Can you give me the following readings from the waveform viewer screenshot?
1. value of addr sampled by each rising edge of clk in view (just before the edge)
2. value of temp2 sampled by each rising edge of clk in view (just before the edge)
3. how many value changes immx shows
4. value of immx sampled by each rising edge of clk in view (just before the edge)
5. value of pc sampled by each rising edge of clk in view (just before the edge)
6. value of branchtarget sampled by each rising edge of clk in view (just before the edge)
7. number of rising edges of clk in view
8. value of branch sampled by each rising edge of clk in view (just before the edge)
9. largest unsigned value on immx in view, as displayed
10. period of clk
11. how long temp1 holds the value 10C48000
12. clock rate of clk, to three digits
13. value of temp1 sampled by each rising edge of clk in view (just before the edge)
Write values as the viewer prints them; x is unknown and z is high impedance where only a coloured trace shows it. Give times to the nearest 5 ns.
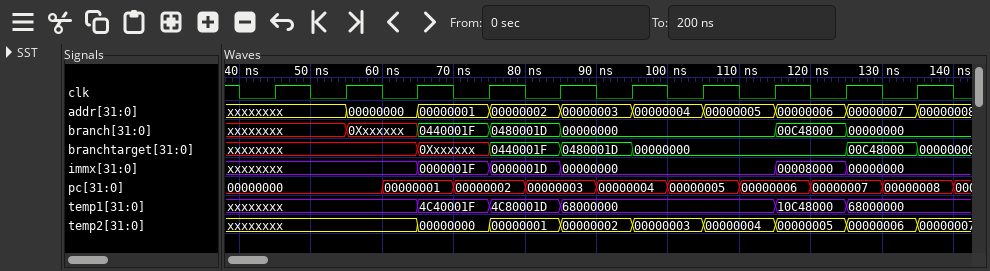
xxxxxxxx, xxxxxxxx, 00000000, 00000001, 00000002, 00000003, 00000004, 00000005, 00000006, 00000007
xxxxxxxx, xxxxxxxx, xxxxxxxx, 00000000, 00000001, 00000002, 00000003, 00000004, 00000005, 00000006
5
xxxxxxxx, xxxxxxxx, xxxxxxxx, 0000001F, 0000001D, 00000000, 00000000, 00000000, 00008000, 00000000
00000000, 00000000, 00000001, 00000002, 00000003, 00000004, 00000005, 00000006, 00000007, 00000008
xxxxxxxx, xxxxxxxx, xxxxxxxx, 0Xxxxxxx, 0440001F, 0480001D, 00000000, 00000000, 00000000, 00C48000
10
xxxxxxxx, xxxxxxxx, 0Xxxxxxx, 0440001F, 0480001D, 00000000, 00000000, 00000000, 00C48000, 00000000
00008000
10 ns
10 ns
100 MHz
xxxxxxxx, xxxxxxxx, xxxxxxxx, 4C40001F, 4C80001D, 68000000, 68000000, 68000000, 10C48000, 68000000
